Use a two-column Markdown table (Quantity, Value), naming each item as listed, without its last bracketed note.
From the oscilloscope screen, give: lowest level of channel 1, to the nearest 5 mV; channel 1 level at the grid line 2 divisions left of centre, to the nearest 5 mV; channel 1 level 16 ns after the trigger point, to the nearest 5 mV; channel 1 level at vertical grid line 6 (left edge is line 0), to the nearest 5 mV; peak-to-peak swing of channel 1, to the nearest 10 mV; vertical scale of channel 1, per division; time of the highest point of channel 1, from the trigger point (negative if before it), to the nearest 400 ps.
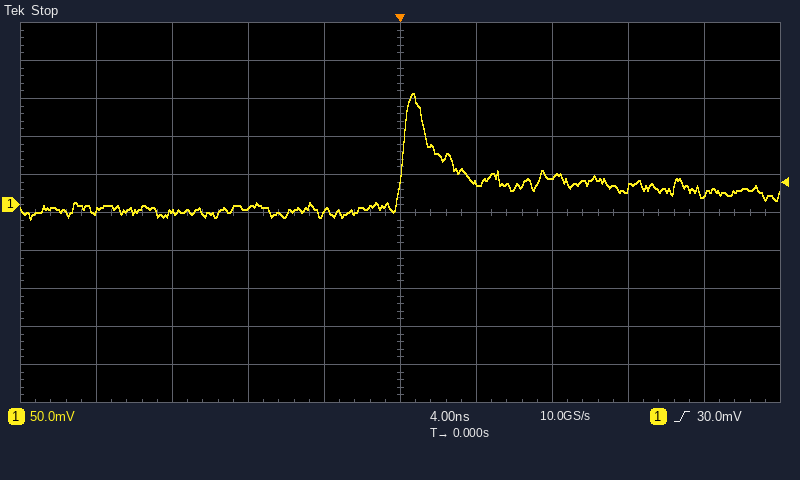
| Quantity | Value |
|---|---|
| lowest level of channel 1, to the nearest 5 mV | -20 mV |
| channel 1 level at the grid line 2 divisions left of centre, to the nearest 5 mV | -5 mV |
| channel 1 level 16 ns after the trigger point, to the nearest 5 mV | 15 mV |
| channel 1 level at vertical grid line 6 (left edge is line 0), to the nearest 5 mV | 30 mV |
| peak-to-peak swing of channel 1, to the nearest 10 mV | 170 mV |
| vertical scale of channel 1, per division | 50 mV |
| time of the highest point of channel 1, from the trigger point (negative if before it), to the nearest 400 ps | +800 ps |
